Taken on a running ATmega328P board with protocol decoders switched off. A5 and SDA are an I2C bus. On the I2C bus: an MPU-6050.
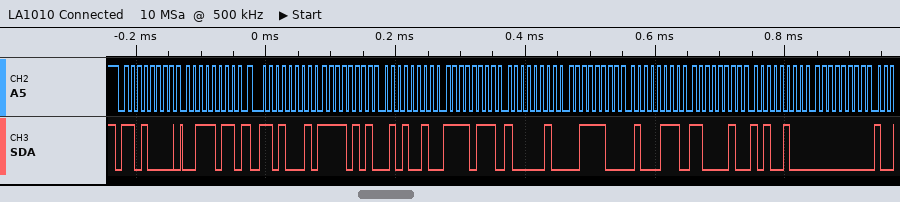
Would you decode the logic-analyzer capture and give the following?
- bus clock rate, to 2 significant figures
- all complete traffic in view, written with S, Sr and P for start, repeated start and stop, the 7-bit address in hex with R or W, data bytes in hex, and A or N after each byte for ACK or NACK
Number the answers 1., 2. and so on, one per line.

1. 100 kHz
2. S 68W A 3B A Sr 68R A F5 A 52 A F7 A 82 A 3C A 47 A C2 A A4 A 00 A
